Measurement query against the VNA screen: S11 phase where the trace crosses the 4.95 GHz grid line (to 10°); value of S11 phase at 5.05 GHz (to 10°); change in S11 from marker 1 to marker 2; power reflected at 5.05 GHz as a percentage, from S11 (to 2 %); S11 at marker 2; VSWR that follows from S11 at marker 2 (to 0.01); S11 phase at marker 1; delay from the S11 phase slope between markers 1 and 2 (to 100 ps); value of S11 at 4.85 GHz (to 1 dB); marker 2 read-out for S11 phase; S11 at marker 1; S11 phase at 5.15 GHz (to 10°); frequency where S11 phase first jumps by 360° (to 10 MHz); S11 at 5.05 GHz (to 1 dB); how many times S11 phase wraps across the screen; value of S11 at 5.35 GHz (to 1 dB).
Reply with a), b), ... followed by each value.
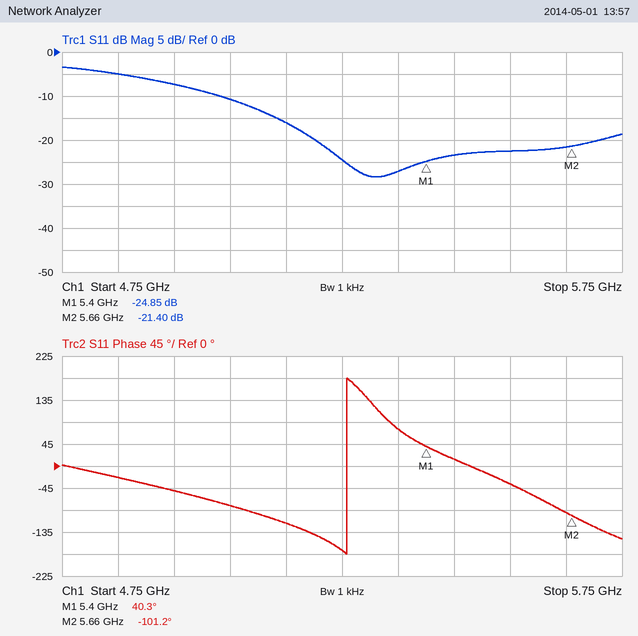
a) -50°
b) -80°
c) 3.45 dB
d) 8 %
e) -21.40 dB
f) 1.19
g) 40.3°
h) 1.5 ns
i) -5 dB
j) -101.2°
k) -24.85 dB
l) -120°
m) 5.26 GHz
n) -11 dB
o) 1
p) -27 dB
